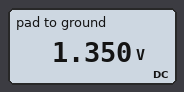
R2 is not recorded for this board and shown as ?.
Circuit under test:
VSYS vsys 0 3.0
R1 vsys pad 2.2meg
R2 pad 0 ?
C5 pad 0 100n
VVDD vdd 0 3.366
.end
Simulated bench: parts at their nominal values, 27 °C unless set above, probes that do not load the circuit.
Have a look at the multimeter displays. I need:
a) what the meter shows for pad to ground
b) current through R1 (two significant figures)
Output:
1.350 V
750 nA
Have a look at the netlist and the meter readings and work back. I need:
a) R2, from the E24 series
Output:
1.8 MΩ
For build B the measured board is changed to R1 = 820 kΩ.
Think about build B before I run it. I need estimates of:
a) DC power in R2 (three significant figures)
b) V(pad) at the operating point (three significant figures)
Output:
2.36 µW
2.06 V
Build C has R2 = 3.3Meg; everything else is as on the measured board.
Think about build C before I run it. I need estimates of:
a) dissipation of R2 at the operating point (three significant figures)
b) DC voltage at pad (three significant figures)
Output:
982 nW
1.80 V
